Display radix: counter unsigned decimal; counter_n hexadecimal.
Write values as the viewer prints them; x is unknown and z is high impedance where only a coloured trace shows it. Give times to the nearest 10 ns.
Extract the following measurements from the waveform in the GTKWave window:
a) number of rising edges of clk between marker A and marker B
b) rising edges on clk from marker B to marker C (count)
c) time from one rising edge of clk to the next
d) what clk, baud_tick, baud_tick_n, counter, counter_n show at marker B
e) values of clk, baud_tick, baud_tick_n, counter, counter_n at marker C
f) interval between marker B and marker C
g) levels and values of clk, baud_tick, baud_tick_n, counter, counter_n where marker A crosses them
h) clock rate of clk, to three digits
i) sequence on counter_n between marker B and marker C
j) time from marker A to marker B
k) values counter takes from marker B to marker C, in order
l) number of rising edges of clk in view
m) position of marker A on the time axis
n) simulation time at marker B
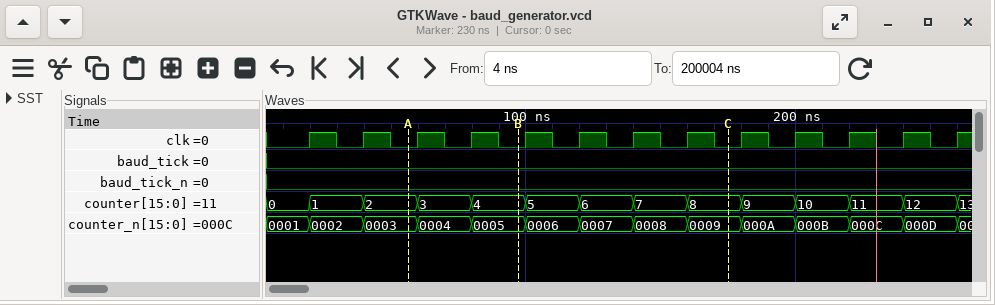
2
4
20 ns
clk=0, baud_tick=0, baud_tick_n=0, counter=4, counter_n=0005
clk=0, baud_tick=0, baud_tick_n=0, counter=8, counter_n=0009
80 ns
clk=0, baud_tick=0, baud_tick_n=0, counter=2, counter_n=0003
50.0 MHz
0005, 0006, 0007, 0008, 0009
40 ns
4, 5, 6, 7, 8
13
60 ns
100 ns
